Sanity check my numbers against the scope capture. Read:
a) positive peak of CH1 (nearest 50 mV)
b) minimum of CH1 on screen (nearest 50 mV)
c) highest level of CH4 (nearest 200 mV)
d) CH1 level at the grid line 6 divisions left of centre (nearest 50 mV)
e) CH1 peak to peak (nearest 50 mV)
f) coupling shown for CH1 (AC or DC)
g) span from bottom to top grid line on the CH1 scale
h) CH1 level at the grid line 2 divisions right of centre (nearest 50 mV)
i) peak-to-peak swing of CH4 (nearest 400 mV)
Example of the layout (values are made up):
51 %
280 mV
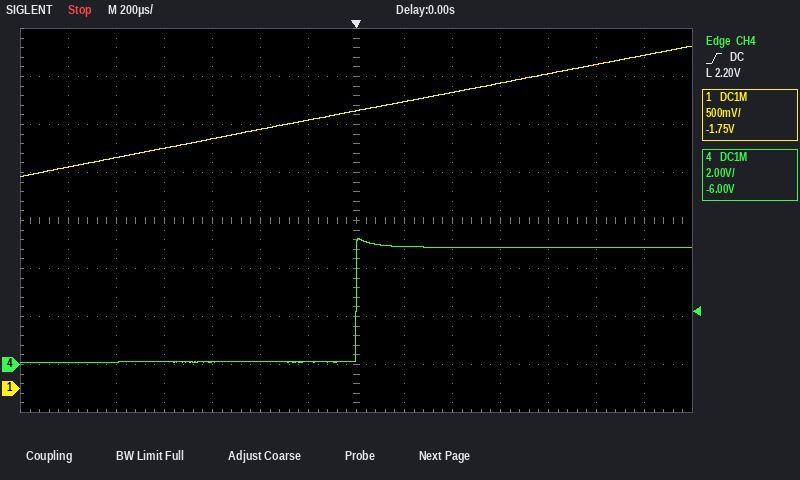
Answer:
3.55 V
2.20 V
5.2 V
2.30 V
1.35 V
DC
4 V
3.10 V
5.2 V
